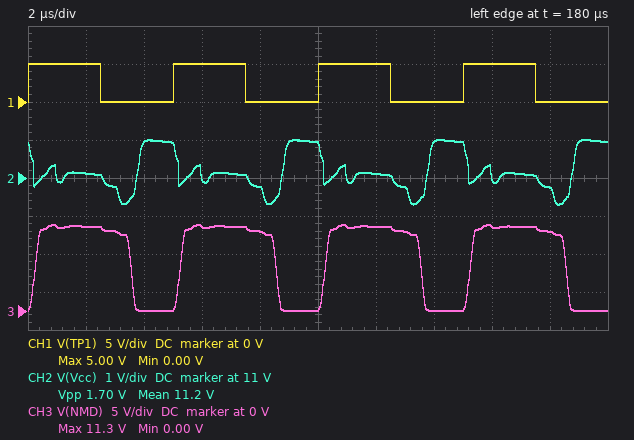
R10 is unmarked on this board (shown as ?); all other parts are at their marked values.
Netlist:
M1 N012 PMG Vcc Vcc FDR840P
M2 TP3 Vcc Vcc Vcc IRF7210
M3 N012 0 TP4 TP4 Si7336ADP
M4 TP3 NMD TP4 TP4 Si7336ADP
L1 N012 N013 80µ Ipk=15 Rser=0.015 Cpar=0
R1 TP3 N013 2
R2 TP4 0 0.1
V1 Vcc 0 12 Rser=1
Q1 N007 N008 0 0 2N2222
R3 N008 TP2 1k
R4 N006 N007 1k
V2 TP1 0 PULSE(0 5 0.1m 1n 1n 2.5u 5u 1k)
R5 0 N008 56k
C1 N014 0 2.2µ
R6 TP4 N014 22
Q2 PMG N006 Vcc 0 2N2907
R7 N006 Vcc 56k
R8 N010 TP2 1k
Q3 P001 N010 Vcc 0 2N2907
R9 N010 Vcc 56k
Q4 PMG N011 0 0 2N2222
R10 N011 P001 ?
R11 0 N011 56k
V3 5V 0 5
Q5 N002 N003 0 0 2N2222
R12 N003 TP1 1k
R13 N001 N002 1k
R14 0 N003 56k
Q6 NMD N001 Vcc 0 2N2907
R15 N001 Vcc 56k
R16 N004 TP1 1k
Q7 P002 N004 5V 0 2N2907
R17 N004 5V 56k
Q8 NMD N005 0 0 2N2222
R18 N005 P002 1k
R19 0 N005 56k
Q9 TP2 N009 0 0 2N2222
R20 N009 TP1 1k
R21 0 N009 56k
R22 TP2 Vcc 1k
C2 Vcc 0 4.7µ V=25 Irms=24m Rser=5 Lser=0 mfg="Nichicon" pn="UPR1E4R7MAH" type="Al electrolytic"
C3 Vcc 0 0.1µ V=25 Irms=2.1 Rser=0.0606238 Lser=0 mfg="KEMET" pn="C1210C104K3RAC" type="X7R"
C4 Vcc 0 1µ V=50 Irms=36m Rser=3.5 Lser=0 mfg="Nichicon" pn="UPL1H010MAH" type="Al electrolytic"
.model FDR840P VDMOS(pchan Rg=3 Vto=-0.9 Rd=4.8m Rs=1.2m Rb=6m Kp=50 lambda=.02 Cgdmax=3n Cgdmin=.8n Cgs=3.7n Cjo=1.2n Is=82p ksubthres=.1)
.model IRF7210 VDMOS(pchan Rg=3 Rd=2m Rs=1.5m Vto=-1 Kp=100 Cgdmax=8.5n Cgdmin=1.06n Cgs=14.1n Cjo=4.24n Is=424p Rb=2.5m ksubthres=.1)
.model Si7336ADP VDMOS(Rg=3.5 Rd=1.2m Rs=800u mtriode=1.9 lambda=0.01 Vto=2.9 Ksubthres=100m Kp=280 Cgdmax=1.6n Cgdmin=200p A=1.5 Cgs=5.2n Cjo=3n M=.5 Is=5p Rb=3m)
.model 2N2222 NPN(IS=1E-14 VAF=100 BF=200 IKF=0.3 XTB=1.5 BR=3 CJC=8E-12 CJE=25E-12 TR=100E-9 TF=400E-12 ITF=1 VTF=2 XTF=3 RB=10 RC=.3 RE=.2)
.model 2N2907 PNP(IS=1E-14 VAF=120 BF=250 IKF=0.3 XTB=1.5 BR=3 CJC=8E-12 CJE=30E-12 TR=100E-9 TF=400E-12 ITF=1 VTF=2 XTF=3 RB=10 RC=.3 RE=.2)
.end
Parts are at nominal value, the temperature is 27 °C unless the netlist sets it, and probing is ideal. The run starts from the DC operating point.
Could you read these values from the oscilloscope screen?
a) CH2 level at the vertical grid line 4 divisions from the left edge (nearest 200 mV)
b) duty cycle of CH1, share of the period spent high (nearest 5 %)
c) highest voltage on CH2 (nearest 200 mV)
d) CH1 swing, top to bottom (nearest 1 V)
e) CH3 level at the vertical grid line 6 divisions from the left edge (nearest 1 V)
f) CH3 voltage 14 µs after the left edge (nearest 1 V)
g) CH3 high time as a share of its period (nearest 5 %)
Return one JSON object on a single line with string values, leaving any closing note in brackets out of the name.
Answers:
{"CH2 level at the vertical grid line 4 divisions from the left edge": "10.8 V", "duty cycle of CH1, share of the period spent high": "50 %", "highest voltage on CH2": "12.0 V", "CH1 swing, top to bottom": "5 V", "CH3 level at the vertical grid line 6 divisions from the left edge": "11 V", "CH3 voltage 14 µs after the left edge": "0 V", "CH3 high time as a share of its period": "65 %"}
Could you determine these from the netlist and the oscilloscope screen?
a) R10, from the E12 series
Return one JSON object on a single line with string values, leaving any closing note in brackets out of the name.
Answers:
{"R10, from the E12 series": "1.5 kΩ"}
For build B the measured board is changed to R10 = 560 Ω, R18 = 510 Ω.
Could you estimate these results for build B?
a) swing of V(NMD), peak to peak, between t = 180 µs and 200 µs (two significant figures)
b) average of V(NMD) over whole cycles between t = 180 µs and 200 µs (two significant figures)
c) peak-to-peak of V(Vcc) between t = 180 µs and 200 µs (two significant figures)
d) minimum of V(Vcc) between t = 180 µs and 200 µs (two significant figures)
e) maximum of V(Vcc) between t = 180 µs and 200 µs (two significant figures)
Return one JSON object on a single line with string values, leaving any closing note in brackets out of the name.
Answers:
{"swing of V(NMD), peak to peak, between t = 180 µs and 200 µs": "9.8 V", "average of V(NMD) over whole cycles between t = 180 µs and 200 µs": "5.3 V", "peak-to-peak of V(Vcc) between t = 180 µs and 200 µs": "2.0 V", "minimum of V(Vcc) between t = 180 µs and 200 µs": "8.9 V", "maximum of V(Vcc) between t = 180 µs and 200 µs": "11 V"}
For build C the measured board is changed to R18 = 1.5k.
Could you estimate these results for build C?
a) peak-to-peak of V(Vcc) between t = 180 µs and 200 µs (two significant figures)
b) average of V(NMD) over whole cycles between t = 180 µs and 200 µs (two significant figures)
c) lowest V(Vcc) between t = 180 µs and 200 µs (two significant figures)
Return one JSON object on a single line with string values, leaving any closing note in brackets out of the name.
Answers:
{"peak-to-peak of V(Vcc) between t = 180 µs and 200 µs": "1.8 V", "average of V(NMD) over whole cycles between t = 180 µs and 200 µs": "7.6 V", "lowest V(Vcc) between t = 180 µs and 200 µs": "10 V"}
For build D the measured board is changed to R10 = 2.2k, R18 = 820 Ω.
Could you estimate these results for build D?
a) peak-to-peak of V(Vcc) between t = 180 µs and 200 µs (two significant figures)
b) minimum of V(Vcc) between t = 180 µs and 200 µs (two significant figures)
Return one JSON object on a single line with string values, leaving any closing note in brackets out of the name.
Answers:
{"peak-to-peak of V(Vcc) between t = 180 µs and 200 µs": "1.3 V", "minimum of V(Vcc) between t = 180 µs and 200 µs": "11 V"}
